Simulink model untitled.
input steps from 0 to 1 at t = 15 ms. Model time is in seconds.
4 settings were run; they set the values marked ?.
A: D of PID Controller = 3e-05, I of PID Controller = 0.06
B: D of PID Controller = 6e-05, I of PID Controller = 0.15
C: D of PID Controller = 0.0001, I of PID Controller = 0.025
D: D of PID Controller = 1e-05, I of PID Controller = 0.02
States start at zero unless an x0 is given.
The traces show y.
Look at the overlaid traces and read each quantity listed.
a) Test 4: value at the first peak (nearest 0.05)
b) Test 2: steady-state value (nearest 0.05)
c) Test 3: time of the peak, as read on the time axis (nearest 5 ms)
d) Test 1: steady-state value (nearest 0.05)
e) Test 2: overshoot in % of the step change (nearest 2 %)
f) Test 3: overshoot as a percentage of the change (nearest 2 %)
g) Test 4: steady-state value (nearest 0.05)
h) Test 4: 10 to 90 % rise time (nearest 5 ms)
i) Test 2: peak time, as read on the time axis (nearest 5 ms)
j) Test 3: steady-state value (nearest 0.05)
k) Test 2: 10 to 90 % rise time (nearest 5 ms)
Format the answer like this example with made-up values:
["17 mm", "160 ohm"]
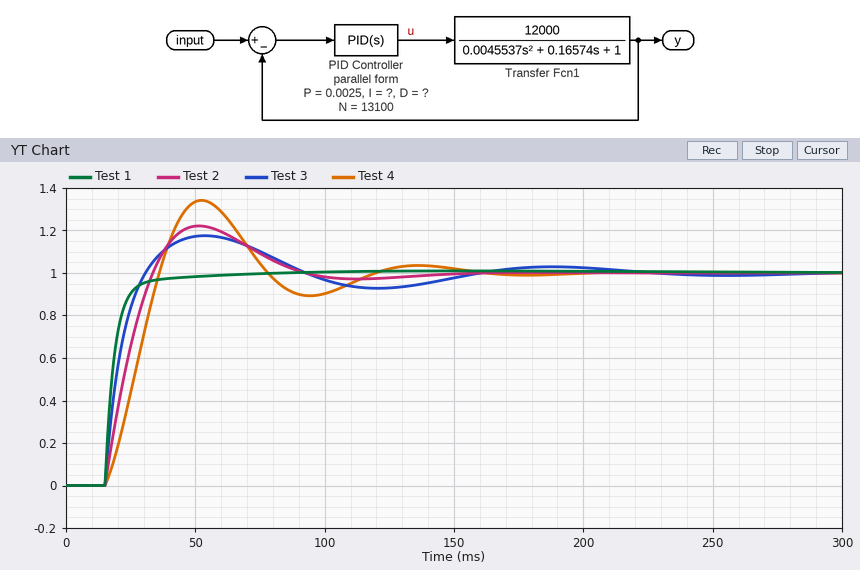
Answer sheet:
["1.35", "1.00", "55 ms", "1.00", "22 %", "18 %", "1.00", "15 ms", "50 ms", "1.00", "15 ms"]
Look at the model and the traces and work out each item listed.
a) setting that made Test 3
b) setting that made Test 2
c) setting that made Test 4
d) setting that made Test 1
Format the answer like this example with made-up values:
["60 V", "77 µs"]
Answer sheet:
["B", "A", "D", "C"]
